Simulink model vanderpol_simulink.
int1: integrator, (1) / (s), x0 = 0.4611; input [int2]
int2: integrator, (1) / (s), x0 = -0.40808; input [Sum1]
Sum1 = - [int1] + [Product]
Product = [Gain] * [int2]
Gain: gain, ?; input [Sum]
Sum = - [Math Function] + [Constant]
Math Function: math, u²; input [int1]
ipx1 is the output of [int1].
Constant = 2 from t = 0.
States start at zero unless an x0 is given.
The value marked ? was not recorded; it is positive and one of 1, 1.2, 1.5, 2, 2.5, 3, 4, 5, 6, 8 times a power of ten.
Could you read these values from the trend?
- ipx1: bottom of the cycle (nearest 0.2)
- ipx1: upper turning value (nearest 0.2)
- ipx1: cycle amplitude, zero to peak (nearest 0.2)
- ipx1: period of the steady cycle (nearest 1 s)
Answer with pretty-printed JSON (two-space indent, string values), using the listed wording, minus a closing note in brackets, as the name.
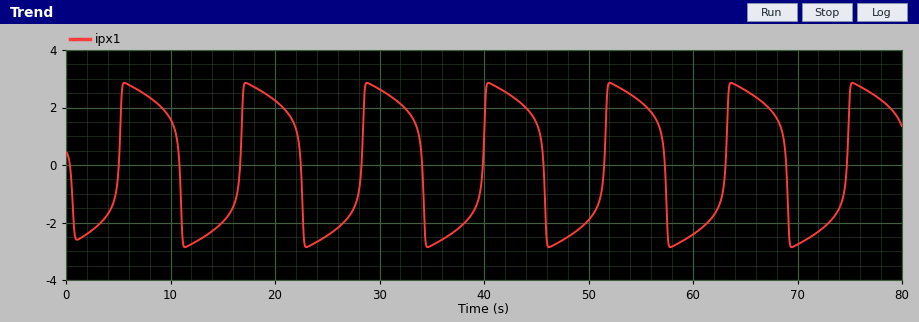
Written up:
{
  "ipx1: bottom of the cycle": "-2.8",
  "ipx1: upper turning value": "2.8",
  "ipx1: cycle amplitude, zero to peak": "2.8",
  "ipx1: period of the steady cycle": "12 s"
}
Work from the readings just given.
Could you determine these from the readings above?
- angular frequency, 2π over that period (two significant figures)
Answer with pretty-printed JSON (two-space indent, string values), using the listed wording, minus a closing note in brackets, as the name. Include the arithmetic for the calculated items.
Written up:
{
  "angular frequency, 2π over that period": "2π / 12 = 0.52 rad/s"
}
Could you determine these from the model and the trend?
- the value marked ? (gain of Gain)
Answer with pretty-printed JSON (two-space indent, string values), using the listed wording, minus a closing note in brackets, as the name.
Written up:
{
  "the value marked ?": "2.5"
}
